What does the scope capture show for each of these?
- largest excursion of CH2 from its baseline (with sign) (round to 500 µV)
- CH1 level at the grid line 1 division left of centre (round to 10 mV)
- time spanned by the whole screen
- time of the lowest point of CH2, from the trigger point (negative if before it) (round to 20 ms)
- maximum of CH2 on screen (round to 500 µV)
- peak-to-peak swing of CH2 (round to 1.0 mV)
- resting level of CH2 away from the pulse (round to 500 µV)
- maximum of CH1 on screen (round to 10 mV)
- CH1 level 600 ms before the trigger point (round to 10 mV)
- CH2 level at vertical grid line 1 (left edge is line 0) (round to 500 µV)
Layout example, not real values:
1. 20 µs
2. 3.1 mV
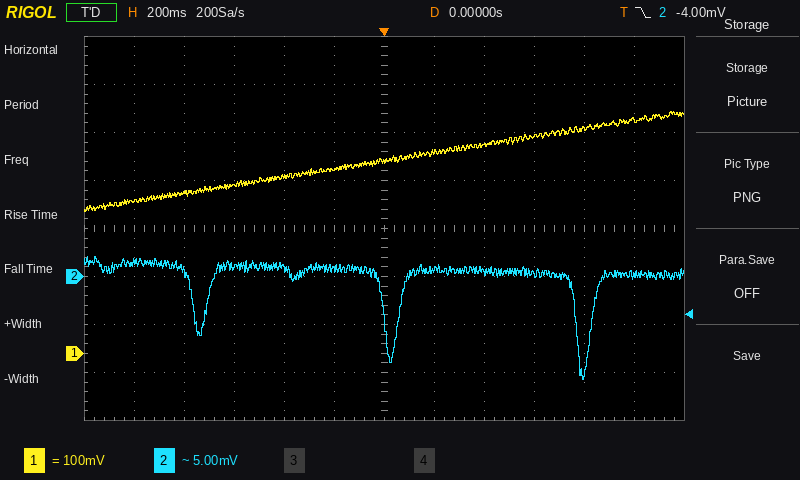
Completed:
1. -11.5 mV
2. 380 mV
3. 2.4 s
4. +800 ms
5. 2.0 mV
6. 13.0 mV
7. 500 µV
8. 500 mV
9. 350 mV
10. 1.5 mV
